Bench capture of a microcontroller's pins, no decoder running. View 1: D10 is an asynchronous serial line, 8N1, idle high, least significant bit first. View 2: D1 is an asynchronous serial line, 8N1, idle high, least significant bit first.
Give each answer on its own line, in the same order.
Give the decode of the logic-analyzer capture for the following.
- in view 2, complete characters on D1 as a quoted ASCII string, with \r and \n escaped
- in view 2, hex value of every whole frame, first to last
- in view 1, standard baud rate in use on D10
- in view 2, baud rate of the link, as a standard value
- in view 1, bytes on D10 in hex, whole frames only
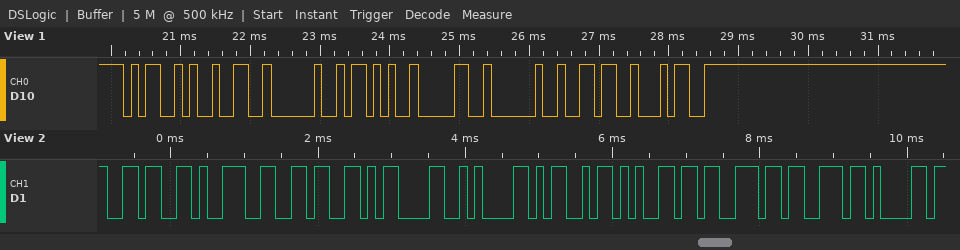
"696\r\nMessa"
36 39 36 0D 0A 4D 65 73 73 61
9600 baud
9600 baud
4D 32 20 2B 30 20 36 34
